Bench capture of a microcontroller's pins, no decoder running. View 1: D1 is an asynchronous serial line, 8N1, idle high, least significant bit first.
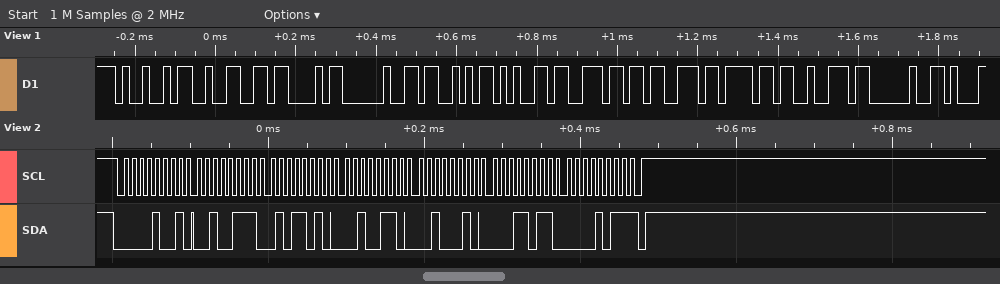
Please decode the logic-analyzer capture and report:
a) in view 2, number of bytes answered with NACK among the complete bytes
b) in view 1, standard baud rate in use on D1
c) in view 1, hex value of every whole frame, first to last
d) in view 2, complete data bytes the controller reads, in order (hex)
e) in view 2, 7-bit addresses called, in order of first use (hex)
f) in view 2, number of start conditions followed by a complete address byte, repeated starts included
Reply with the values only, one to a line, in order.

1
57600 baud
49 32 43 20 53 65 6E 73 6F 72 20
27 5A 26 22 1B 0B
0x04
1
